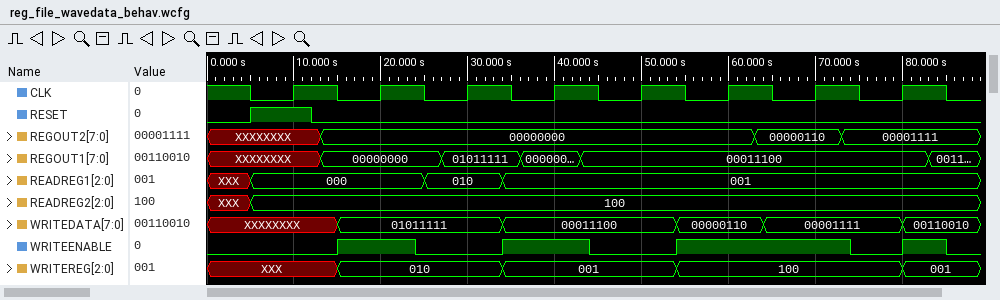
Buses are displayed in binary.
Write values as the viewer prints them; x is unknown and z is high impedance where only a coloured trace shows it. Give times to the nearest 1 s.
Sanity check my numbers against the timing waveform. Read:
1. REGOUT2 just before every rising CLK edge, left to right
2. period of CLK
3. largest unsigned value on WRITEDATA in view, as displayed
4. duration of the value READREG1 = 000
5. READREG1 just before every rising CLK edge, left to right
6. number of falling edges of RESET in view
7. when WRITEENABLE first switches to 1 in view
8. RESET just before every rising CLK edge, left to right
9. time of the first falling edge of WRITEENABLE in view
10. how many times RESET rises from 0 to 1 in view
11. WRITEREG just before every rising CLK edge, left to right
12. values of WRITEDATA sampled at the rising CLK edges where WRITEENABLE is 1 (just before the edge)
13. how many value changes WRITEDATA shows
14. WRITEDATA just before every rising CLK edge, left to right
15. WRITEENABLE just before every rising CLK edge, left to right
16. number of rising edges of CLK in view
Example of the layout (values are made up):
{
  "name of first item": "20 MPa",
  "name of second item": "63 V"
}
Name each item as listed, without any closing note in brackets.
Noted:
{
  "REGOUT2 just before every rising CLK edge, left to right": "XXXXXXXX, 00000000, 00000000, 00000000, 00000000, 00000000, 00000110, 00001111",
  "period of CLK": "10 s",
  "largest unsigned value on WRITEDATA in view, as displayed": "01011111",
  "duration of the value READREG1 = 000": "20 s",
  "READREG1 just before every rising CLK edge, left to right": "000, 000, 010, 001, 001, 001, 001, 001",
  "number of falling edges of RESET in view": "1",
  "when WRITEENABLE first switches to 1 in view": "15 s",
  "RESET just before every rising CLK edge, left to right": "1 0 0 0 0 0 0 0",
  "time of the first falling edge of WRITEENABLE in view": "24 s",
  "how many times RESET rises from 0 to 1 in view": "1",
  "WRITEREG just before every rising CLK edge, left to right": "XXX, 010, 010, 001, 001, 100, 100, 100",
  "values of WRITEDATA sampled at the rising CLK edges where WRITEENABLE is 1": "01011111, 00011100, 00000110, 00001111",
  "how many value changes WRITEDATA shows": "5",
  "WRITEDATA just before every rising CLK edge, left to right": "XXXXXXXX, 01011111, 01011111, 00011100, 00011100, 00000110, 00001111, 00001111",
  "WRITEENABLE just before every rising CLK edge, left to right": "0 1 0 1 0 1 1 0",
  "number of rising edges of CLK in view": "8"
}
